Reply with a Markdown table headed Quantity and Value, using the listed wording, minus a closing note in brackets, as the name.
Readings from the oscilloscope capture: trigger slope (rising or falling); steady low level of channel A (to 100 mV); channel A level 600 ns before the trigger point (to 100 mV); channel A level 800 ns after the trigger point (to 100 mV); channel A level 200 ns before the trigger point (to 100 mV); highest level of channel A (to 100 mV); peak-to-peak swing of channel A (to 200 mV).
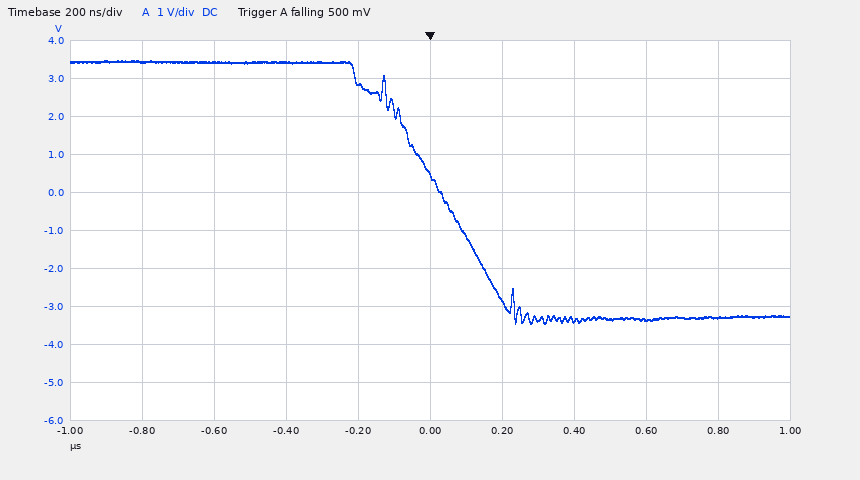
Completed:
| Quantity | Value |
|---|---|
| trigger slope | falling |
| steady low level of channel A | -3.3 V |
| channel A level 600 ns before the trigger point | 3.4 V |
| channel A level 800 ns after the trigger point | -3.3 V |
| channel A level 200 ns before the trigger point | 2.9 V |
| highest level of channel A | 3.5 V |
| peak-to-peak swing of channel A | 7.0 V |
